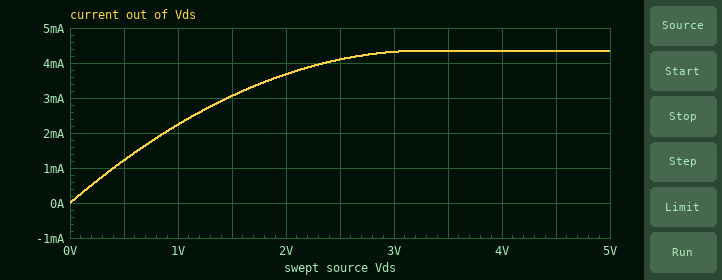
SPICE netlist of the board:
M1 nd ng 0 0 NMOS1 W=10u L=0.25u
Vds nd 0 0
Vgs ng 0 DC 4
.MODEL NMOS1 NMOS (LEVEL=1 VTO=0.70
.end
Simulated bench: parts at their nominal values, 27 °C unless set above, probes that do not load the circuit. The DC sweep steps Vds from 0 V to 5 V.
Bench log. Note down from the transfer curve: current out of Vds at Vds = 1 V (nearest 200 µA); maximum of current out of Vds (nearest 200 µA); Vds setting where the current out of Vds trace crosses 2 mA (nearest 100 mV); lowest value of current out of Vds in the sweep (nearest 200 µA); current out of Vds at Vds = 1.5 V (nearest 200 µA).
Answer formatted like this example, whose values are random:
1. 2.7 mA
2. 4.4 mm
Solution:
1. 2.2 mA
2. 4.4 mA
3. 900 mV
4. 0 A
5. 3.0 mA
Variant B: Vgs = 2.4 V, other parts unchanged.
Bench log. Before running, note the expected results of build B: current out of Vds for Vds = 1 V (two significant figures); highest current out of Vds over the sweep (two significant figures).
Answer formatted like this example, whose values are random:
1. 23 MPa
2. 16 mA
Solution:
1. 960 µA
2. 1.2 mA
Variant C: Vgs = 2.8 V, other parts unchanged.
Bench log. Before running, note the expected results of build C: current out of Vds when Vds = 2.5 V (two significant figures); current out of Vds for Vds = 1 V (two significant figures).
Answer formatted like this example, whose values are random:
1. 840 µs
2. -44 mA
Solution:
1. 1.8 mA
2. 1.3 mA
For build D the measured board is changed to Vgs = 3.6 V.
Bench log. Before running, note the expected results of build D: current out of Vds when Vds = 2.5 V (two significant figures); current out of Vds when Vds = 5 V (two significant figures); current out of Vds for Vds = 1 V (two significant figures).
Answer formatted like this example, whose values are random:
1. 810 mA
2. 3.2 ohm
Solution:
1. 3.3 mA
2. 3.4 mA
3. 1.9 mA
